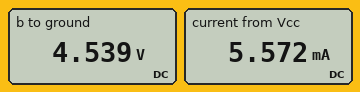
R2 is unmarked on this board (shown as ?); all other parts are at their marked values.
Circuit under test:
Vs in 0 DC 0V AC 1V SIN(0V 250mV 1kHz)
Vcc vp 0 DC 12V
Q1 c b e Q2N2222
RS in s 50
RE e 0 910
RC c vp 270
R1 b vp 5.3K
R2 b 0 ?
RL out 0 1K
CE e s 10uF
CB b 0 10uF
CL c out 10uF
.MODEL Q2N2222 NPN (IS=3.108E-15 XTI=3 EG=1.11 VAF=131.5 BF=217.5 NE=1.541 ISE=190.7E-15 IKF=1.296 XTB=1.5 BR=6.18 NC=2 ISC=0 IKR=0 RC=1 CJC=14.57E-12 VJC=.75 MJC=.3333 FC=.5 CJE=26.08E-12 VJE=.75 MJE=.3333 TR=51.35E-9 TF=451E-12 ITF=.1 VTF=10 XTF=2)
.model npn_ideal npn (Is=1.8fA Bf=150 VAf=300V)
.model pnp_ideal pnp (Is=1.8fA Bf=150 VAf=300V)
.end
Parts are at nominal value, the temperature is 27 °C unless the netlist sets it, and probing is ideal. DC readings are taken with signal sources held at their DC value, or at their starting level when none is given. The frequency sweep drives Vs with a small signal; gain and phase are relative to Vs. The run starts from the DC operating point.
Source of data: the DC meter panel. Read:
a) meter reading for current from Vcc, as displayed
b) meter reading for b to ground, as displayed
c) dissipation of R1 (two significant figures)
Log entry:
5.572 mA
4.539 V
11 mW
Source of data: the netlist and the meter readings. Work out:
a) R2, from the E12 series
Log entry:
3.3 kΩ
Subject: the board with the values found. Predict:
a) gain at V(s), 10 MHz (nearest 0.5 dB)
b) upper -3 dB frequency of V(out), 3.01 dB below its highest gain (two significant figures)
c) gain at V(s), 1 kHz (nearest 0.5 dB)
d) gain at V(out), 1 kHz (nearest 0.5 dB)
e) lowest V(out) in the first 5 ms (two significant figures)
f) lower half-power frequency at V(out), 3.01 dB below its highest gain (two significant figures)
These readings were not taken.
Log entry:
-19.0 dB
94 MHz
-10.5 dB
11.0 dB
-990 mV
290 Hz
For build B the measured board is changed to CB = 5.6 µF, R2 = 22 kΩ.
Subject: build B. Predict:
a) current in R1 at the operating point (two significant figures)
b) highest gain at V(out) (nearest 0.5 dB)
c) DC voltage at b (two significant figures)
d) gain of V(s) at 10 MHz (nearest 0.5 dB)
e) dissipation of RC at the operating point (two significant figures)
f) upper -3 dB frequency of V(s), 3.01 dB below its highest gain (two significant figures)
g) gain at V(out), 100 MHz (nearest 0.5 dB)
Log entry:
490 µA
12.0 dB
9.4 V
-25.5 dB
24 mW
310 Hz
5.0 dB
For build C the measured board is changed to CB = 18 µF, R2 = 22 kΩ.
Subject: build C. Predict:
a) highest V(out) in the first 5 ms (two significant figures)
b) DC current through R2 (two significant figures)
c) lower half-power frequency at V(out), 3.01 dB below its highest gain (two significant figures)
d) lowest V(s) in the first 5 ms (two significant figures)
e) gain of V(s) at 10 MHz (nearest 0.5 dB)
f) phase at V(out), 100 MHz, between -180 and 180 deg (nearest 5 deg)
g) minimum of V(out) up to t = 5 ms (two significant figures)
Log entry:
940 mV
430 µA
300 Hz
-77 mV
-25.5 dB
-80 deg
-810 mV
